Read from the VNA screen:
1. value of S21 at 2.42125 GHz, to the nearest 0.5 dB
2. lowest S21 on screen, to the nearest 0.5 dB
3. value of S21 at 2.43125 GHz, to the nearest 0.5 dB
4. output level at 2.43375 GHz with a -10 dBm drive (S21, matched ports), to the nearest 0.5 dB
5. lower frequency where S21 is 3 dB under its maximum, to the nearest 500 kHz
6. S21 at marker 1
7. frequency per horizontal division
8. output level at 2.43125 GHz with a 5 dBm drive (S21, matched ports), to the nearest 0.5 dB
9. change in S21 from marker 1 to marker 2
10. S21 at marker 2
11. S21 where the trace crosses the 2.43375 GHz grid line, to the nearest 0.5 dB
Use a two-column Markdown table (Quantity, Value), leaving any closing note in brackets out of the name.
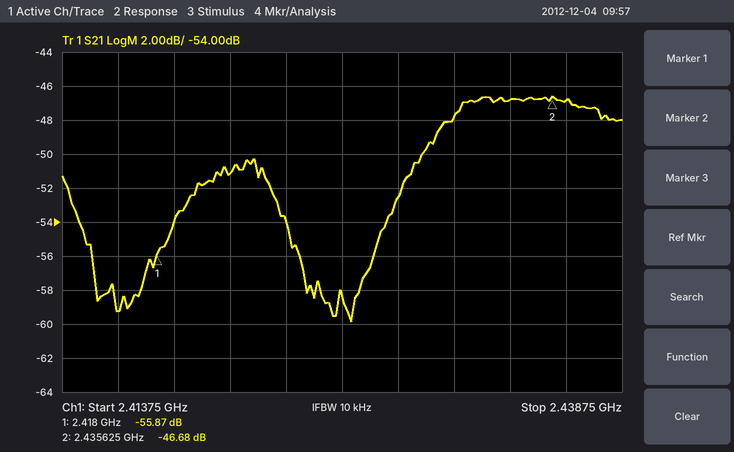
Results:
| Quantity | Value |
|---|---|
| value of S21 at 2.42125 GHz, to the nearest 0.5 dB | -51.0 dB |
| lowest S21 on screen, to the nearest 0.5 dB | -60.0 dB |
| value of S21 at 2.43125 GHz, to the nearest 0.5 dB | -48.0 dB |
| output level at 2.43375 GHz with a -10 dBm drive (S21, matched ports), to the nearest 0.5 dB | -57.0 dBm |
| lower frequency where S21 is 3 dB under its maximum, to the nearest 500 kHz | 2.4300 GHz |
| S21 at marker 1 | -55.87 dB |
| frequency per horizontal division | 2.5 MHz |
| output level at 2.43125 GHz with a 5 dBm drive (S21, matched ports), to the nearest 0.5 dB | -43.0 dBm |
| change in S21 from marker 1 to marker 2 | 9.19 dB |
| S21 at marker 2 | -46.68 dB |
| S21 where the trace crosses the 2.43375 GHz grid line, to the nearest 0.5 dB | -47.0 dB |
